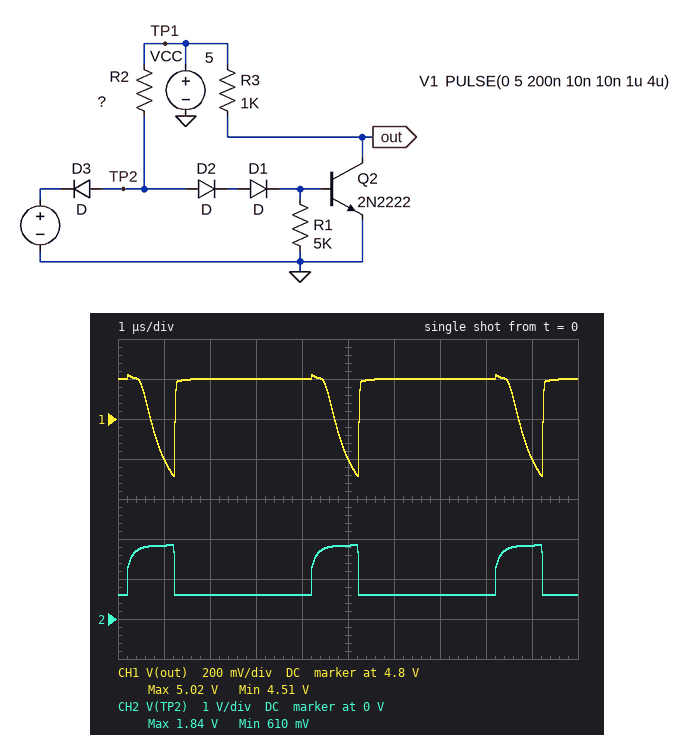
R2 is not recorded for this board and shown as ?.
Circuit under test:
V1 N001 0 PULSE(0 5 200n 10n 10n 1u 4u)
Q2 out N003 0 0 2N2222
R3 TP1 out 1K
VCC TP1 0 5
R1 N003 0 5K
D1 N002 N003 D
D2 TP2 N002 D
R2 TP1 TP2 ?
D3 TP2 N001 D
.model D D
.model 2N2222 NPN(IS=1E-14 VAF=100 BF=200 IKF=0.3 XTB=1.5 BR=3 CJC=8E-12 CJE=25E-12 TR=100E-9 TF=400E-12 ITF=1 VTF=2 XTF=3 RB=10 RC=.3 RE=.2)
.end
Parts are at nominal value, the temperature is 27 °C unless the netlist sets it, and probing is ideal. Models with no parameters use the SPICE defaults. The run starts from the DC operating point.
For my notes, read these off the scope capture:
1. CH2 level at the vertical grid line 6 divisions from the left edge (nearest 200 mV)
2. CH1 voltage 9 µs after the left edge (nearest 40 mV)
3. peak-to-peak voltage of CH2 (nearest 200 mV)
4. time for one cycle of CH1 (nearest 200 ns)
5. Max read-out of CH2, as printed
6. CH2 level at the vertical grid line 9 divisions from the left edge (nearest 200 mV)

600 mV
4.60 V
1.2 V
4.0 µs
1.84 V
1.8 V
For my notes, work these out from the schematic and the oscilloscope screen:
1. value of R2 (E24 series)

24 kΩ
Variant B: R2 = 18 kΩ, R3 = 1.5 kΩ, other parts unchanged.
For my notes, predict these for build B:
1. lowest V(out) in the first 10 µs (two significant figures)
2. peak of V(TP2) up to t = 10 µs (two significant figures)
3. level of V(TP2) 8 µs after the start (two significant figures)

830 mV
1.9 V
620 mV
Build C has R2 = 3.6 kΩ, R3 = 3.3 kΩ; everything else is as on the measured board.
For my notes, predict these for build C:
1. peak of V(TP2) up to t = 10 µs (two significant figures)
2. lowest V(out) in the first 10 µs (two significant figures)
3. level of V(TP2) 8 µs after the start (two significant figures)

2.0 V
15 mV
660 mV
